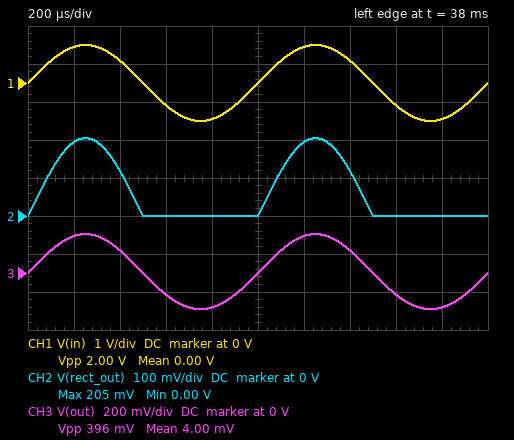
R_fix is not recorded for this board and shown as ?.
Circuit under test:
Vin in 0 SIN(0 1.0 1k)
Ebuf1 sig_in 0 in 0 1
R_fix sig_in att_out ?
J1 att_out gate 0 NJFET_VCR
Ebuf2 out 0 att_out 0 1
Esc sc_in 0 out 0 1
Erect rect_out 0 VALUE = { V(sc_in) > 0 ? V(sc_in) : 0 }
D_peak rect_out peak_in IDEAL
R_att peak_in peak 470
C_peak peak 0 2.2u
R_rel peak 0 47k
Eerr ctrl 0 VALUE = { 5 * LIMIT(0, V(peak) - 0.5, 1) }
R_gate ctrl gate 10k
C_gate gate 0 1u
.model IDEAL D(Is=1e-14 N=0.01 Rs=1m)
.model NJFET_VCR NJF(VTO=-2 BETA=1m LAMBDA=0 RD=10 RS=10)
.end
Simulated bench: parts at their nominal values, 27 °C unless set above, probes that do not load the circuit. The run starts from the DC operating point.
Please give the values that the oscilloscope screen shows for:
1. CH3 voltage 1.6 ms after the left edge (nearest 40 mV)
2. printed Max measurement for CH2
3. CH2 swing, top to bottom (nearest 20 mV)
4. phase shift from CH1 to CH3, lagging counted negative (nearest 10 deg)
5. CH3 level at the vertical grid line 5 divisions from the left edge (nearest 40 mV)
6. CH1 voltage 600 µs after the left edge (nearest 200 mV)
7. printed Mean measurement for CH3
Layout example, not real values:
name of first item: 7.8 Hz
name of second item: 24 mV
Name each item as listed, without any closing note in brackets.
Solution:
CH3 voltage 1.6 ms after the left edge: -120 mV
printed Max measurement for CH2: 205 mV
CH2 swing, top to bottom: 200 mV
phase shift from CH1 to CH3, lagging counted negative: 0 deg
CH3 level at the vertical grid line 5 divisions from the left edge: 0 V
CH1 voltage 600 µs after the left edge: -600 mV
printed Mean measurement for CH3: 4.00 mV
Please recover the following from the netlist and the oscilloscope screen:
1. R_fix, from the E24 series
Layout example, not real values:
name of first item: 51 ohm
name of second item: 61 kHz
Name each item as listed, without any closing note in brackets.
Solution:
R_fix, from the E24 series: 1.1 kΩ
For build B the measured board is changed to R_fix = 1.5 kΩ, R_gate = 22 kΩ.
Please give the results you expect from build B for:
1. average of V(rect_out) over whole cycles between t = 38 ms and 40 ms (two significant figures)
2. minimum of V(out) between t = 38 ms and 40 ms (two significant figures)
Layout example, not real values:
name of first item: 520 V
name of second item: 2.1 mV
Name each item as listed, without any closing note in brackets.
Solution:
average of V(rect_out) over whole cycles between t = 38 ms and 40 ms: 50 mV
minimum of V(out) between t = 38 ms and 40 ms: -150 mV
